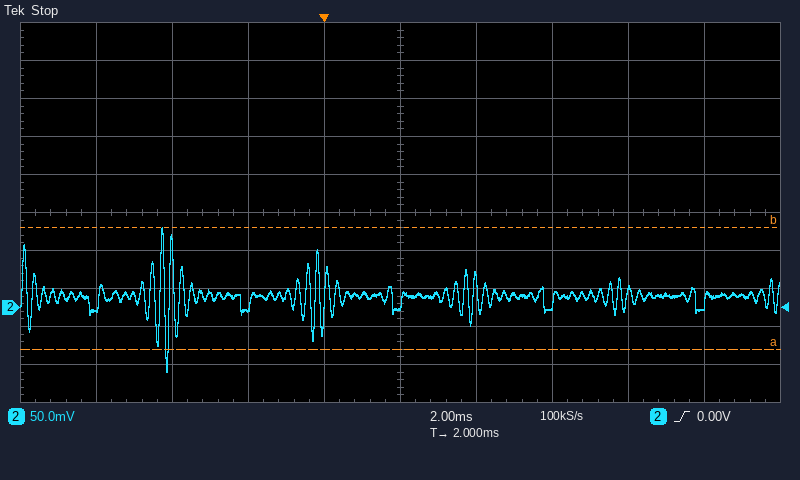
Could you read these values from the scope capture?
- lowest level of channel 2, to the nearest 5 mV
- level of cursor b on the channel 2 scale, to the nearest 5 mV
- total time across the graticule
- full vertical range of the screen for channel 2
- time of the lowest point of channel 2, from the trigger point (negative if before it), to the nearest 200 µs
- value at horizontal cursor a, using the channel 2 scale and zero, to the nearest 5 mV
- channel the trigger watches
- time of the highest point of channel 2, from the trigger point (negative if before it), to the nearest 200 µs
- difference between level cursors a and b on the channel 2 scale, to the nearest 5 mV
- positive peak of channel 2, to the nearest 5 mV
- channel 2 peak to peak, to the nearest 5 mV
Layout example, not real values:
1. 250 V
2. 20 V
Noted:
1. -85 mV
2. 105 mV
3. 20 ms
4. 500 mV
5. -4.2 ms
6. -55 mV
7. channel 2
8. -4.2 ms
9. 160 mV
10. 105 mV
11. 190 mV
